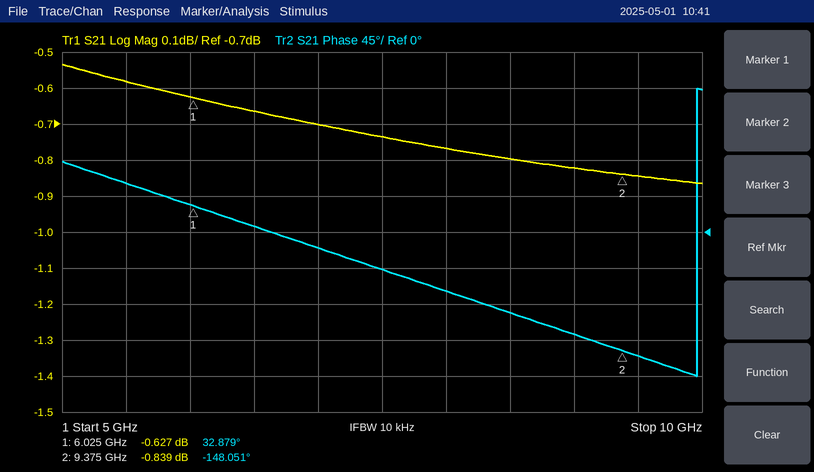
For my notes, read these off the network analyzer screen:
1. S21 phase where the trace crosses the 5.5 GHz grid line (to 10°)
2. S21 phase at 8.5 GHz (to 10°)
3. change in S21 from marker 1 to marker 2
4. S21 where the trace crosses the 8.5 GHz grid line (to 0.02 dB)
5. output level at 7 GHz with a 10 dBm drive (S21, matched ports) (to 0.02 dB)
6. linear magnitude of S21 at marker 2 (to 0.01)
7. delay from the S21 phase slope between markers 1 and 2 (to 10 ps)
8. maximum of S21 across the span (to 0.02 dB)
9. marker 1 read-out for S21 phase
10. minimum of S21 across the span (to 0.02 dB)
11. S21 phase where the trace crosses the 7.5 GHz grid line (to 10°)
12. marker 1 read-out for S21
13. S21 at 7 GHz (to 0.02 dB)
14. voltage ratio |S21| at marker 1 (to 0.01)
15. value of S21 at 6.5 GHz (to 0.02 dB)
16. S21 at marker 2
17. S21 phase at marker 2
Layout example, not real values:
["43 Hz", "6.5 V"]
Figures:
["60°", "-100°", "-0.212 dB", "-0.80 dB", "9.30 dBm", "0.91", "150 ps", "-0.54 dB", "32.879°", "-0.86 dB", "-50°", "-0.627 dB", "-0.70 dB", "0.93", "-0.66 dB", "-0.839 dB", "-148.051°"]
